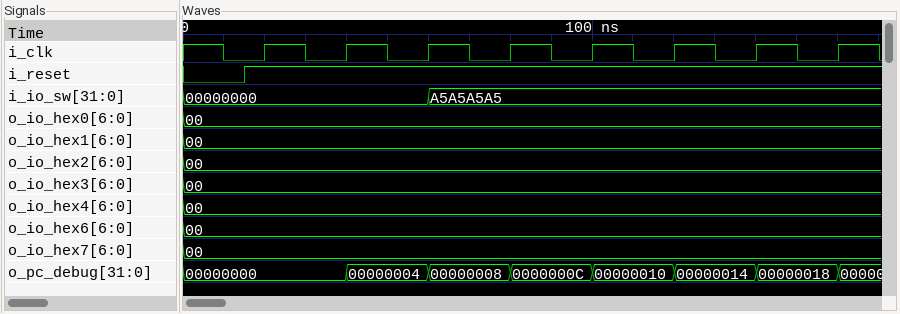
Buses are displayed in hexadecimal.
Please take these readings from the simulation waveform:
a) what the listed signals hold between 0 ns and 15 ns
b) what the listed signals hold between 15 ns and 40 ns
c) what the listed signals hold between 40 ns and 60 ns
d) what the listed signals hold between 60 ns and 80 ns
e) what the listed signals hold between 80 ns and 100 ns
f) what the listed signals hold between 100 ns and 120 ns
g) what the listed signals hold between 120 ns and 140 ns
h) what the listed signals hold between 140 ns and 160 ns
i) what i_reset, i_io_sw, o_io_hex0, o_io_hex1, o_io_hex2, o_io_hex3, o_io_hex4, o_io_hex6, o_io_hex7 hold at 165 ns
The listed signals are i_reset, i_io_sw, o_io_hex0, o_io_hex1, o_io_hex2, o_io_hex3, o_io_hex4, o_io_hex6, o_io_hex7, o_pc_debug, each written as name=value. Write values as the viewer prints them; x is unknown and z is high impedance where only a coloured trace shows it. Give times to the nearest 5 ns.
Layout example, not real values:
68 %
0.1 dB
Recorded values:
i_reset=0, i_io_sw=00000000, o_io_hex0=00, o_io_hex1=00, o_io_hex2=00, o_io_hex3=00, o_io_hex4=00, o_io_hex6=00, o_io_hex7=00, o_pc_debug=00000000
i_reset=1, i_io_sw=00000000, o_io_hex0=00, o_io_hex1=00, o_io_hex2=00, o_io_hex3=00, o_io_hex4=00, o_io_hex6=00, o_io_hex7=00, o_pc_debug=00000000
i_reset=1, i_io_sw=00000000, o_io_hex0=00, o_io_hex1=00, o_io_hex2=00, o_io_hex3=00, o_io_hex4=00, o_io_hex6=00, o_io_hex7=00, o_pc_debug=00000004
i_reset=1, i_io_sw=A5A5A5A5, o_io_hex0=00, o_io_hex1=00, o_io_hex2=00, o_io_hex3=00, o_io_hex4=00, o_io_hex6=00, o_io_hex7=00, o_pc_debug=00000008
i_reset=1, i_io_sw=A5A5A5A5, o_io_hex0=00, o_io_hex1=00, o_io_hex2=00, o_io_hex3=00, o_io_hex4=00, o_io_hex6=00, o_io_hex7=00, o_pc_debug=0000000C
i_reset=1, i_io_sw=A5A5A5A5, o_io_hex0=00, o_io_hex1=00, o_io_hex2=00, o_io_hex3=00, o_io_hex4=00, o_io_hex6=00, o_io_hex7=00, o_pc_debug=00000010
i_reset=1, i_io_sw=A5A5A5A5, o_io_hex0=00, o_io_hex1=00, o_io_hex2=00, o_io_hex3=00, o_io_hex4=00, o_io_hex6=00, o_io_hex7=00, o_pc_debug=00000014
i_reset=1, i_io_sw=A5A5A5A5, o_io_hex0=00, o_io_hex1=00, o_io_hex2=00, o_io_hex3=00, o_io_hex4=00, o_io_hex6=00, o_io_hex7=00, o_pc_debug=00000018
i_reset=1, i_io_sw=A5A5A5A5, o_io_hex0=00, o_io_hex1=00, o_io_hex2=00, o_io_hex3=00, o_io_hex4=00, o_io_hex6=00, o_io_hex7=00
